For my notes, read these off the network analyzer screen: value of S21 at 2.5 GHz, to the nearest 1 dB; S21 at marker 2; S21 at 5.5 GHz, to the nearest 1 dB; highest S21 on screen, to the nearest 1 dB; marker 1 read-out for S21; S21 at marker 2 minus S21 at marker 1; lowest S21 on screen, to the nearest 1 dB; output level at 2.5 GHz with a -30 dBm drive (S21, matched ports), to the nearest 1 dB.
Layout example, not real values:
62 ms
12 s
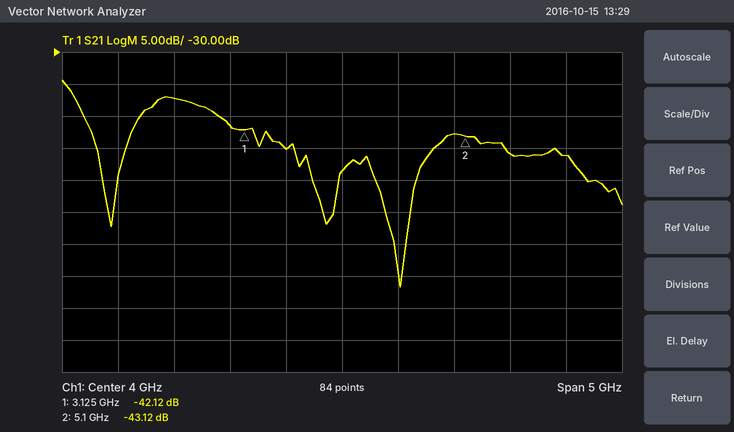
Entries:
-37 dB
-43.12 dB
-46 dB
-34 dB
-42.12 dB
-1.00 dB
-67 dB
-67 dBm
